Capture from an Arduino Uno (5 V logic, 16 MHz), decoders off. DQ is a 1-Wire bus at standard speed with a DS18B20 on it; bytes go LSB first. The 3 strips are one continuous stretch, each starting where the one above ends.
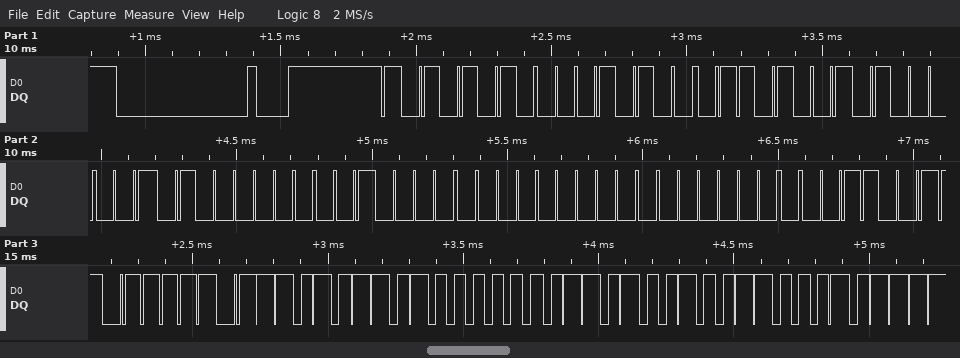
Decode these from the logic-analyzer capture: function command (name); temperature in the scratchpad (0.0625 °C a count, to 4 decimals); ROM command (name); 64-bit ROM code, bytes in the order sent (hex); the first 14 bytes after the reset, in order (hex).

Read Scratchpad
22.6875 °C
Match ROM
28 96 82 02 04 00 00 CC
55 28 96 82 02 04 00 00 CC BE 6B 01 4B 46
